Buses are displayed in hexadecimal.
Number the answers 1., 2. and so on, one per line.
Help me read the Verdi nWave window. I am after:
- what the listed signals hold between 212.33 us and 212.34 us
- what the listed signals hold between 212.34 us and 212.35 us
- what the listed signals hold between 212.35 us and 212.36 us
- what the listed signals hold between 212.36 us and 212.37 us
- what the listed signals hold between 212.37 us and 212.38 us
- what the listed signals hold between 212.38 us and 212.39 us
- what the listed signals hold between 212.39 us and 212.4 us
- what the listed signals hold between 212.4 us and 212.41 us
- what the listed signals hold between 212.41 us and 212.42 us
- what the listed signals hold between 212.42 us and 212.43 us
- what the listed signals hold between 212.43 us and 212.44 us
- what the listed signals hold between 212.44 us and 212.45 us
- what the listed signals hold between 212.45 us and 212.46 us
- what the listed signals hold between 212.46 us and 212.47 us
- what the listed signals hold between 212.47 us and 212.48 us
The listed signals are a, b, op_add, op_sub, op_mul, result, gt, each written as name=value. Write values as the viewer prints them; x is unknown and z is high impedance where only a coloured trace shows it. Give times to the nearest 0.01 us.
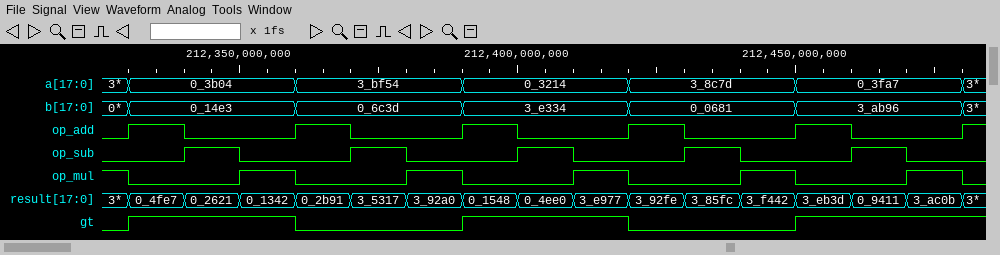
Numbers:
1. a=0_3b04, b=0_14e3, op_add=1, op_sub=0, op_mul=0, result=0_4fe7, gt=1
2. a=0_3b04, b=0_14e3, op_add=0, op_sub=1, op_mul=0, result=0_2621, gt=1
3. a=0_3b04, b=0_14e3, op_add=0, op_sub=0, op_mul=1, result=0_1342, gt=1
4. a=3_bf54, b=0_6c3d, op_add=1, op_sub=0, op_mul=0, result=0_2b91, gt=0
5. a=3_bf54, b=0_6c3d, op_add=0, op_sub=1, op_mul=0, result=3_5317, gt=0
6. a=3_bf54, b=0_6c3d, op_add=0, op_sub=0, op_mul=1, result=3_92a0, gt=0
7. a=0_3214, b=3_e334, op_add=1, op_sub=0, op_mul=0, result=0_1548, gt=1
8. a=0_3214, b=3_e334, op_add=0, op_sub=1, op_mul=0, result=0_4ee0, gt=1
9. a=0_3214, b=3_e334, op_add=0, op_sub=0, op_mul=1, result=3_e977, gt=1
10. a=3_8c7d, b=0_0681, op_add=1, op_sub=0, op_mul=0, result=3_92fe, gt=0
11. a=3_8c7d, b=0_0681, op_add=0, op_sub=1, op_mul=0, result=3_85fc, gt=0
12. a=3_8c7d, b=0_0681, op_add=0, op_sub=0, op_mul=1, result=3_f442, gt=0
13. a=0_3fa7, b=3_ab96, op_add=1, op_sub=0, op_mul=0, result=3_eb3d, gt=1
14. a=0_3fa7, b=3_ab96, op_add=0, op_sub=1, op_mul=0, result=0_9411, gt=1
15. a=0_3fa7, b=3_ab96, op_add=0, op_sub=0, op_mul=1, result=3_ac0b, gt=1
